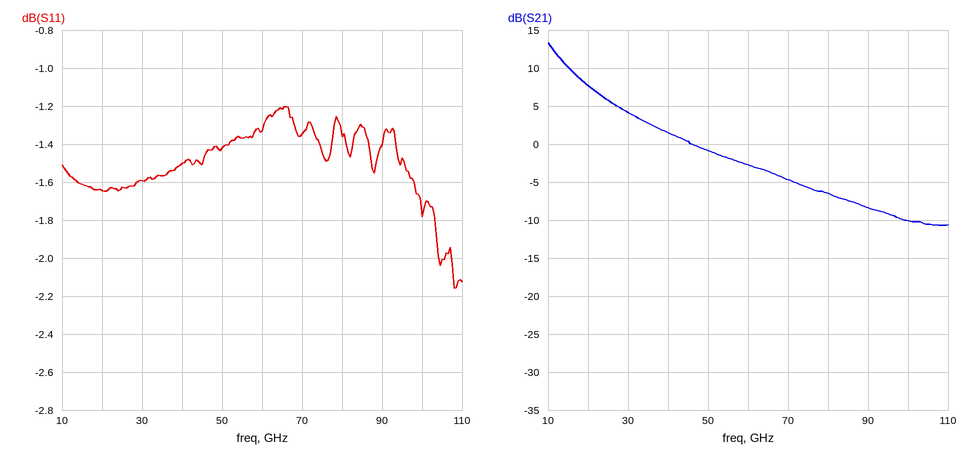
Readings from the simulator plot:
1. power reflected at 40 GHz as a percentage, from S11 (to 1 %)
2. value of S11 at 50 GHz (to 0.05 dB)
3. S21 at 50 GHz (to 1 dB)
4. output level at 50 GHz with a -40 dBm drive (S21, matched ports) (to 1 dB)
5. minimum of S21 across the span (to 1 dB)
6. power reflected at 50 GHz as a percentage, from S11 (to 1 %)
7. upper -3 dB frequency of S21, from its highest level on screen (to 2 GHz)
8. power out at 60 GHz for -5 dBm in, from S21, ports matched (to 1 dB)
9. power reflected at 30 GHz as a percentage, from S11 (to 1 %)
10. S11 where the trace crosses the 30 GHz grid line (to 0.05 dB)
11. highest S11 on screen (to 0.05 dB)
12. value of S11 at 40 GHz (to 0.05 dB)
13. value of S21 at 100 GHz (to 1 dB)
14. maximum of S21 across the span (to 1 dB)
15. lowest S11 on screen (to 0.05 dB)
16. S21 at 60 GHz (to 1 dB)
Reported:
71 %
-1.40 dB
-1 dB
-41 dBm
-11 dB
72 %
14 GHz
-8 dBm
69 %
-1.60 dB
-1.20 dB
-1.50 dB
-10 dB
13 dB
-2.15 dB
-3 dB
